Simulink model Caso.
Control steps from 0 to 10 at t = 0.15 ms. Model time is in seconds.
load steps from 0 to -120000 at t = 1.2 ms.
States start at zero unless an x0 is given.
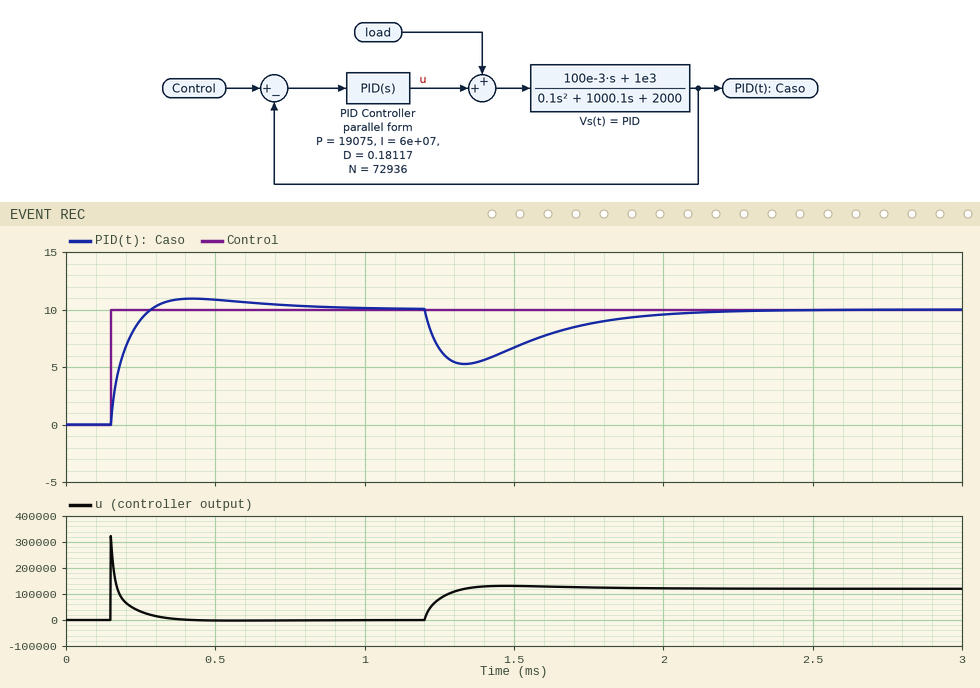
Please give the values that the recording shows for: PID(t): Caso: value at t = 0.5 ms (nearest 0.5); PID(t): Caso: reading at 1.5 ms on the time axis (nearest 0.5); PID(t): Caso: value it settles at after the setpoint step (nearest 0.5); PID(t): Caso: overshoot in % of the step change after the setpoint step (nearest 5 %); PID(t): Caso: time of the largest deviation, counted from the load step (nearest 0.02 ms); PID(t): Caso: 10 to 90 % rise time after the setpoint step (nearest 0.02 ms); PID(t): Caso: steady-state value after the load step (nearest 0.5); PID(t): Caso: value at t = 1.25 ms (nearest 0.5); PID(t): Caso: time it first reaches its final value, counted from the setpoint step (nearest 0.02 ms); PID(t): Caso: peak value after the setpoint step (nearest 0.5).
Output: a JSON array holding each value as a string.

["11.0", "6.5", "10.0", "10 %", "0.14 ms", "0.10 ms", "10.0", "6.5", "0.14 ms", "11.0"]
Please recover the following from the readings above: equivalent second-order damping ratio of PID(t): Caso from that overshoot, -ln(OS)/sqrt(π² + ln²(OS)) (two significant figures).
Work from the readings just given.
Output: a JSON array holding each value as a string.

["0.59"]
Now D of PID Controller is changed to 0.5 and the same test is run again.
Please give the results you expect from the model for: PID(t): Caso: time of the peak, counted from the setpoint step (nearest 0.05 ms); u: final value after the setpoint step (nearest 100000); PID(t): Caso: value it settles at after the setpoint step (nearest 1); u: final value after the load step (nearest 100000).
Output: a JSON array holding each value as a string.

["0.30 ms", "0", "10", "100000"]
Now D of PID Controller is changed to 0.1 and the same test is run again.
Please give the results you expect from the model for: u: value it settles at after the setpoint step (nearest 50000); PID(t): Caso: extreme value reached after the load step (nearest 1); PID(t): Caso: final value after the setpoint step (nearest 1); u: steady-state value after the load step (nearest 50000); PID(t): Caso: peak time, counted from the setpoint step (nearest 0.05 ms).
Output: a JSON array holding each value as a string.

["0", "5", "10", "100000", "0.25 ms"]
